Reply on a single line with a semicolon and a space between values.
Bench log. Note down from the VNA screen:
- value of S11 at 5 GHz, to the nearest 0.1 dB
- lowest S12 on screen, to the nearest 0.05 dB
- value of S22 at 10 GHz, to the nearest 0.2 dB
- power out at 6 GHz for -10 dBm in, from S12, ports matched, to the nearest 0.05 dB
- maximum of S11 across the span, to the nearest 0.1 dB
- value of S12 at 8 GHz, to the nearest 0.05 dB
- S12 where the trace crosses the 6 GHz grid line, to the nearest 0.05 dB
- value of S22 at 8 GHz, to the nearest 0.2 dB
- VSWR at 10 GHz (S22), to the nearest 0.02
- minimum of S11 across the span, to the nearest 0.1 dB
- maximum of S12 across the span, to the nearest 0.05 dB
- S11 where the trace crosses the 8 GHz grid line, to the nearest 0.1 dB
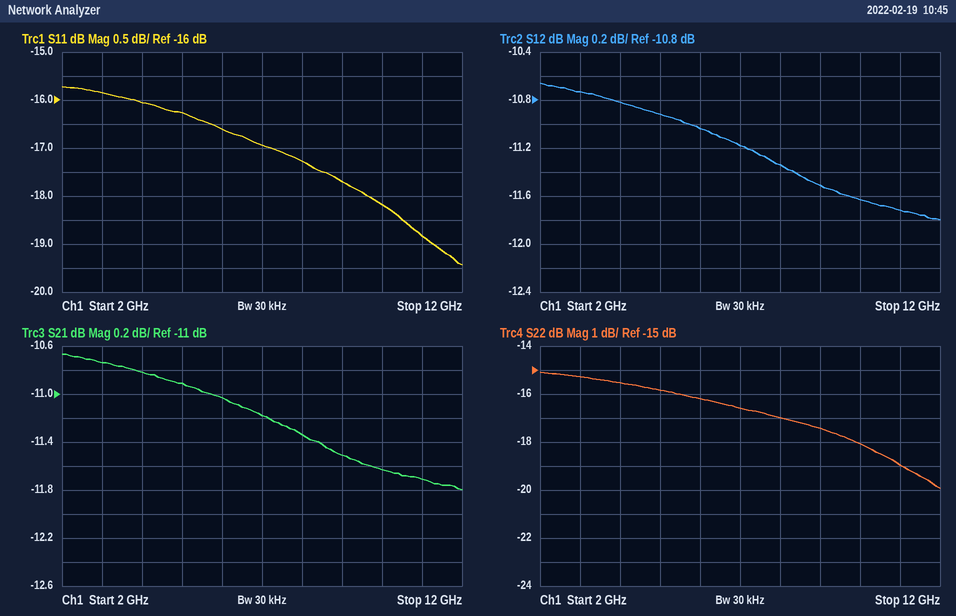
-16.3 dB; -11.80 dB; -18.0 dB; -21.05 dBm; -15.7 dB; -11.35 dB; -11.05 dB; -17.0 dB; 1.28; -19.4 dB; -10.65 dB; -17.3 dB
